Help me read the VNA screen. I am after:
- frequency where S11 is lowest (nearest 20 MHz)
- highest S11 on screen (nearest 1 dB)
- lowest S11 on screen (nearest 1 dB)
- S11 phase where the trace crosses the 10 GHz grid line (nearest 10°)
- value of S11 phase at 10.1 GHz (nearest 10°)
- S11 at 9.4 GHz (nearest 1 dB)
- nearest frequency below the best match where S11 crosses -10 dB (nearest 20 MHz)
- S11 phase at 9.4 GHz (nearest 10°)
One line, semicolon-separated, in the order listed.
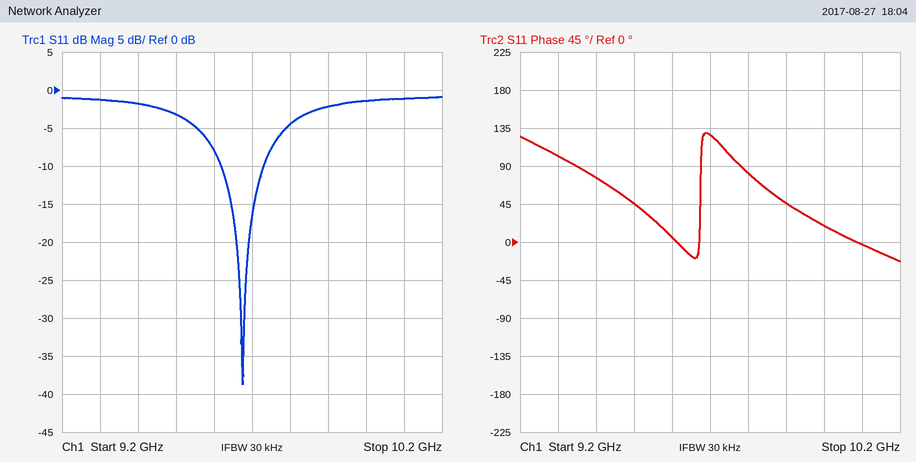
9.68 GHz; -1 dB; -39 dB; 20°; 0°; -2 dB; 9.62 GHz; 80°
